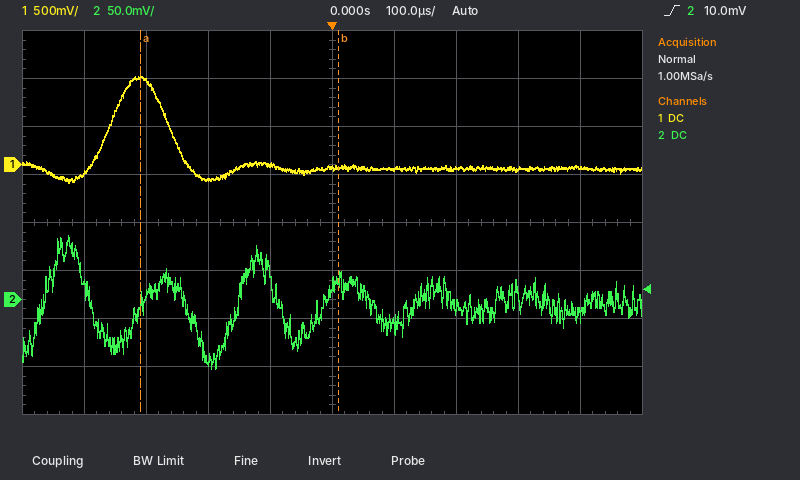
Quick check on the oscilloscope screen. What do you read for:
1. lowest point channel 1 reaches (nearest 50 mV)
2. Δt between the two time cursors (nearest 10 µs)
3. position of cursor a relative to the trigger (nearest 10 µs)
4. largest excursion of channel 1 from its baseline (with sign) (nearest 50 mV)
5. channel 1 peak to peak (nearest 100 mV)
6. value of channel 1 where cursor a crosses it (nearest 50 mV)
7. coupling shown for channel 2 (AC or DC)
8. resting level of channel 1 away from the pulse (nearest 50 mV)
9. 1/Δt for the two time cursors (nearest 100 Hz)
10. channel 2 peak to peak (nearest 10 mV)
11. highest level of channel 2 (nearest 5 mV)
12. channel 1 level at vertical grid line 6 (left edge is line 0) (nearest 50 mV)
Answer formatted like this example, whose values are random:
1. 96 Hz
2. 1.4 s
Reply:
1. -200 mV
2. 320 µs
3. -310 µs
4. +950 mV
5. 1.10 V
6. 900 mV
7. DC
8. -50 mV
9. 3.1 kHz
10. 140 mV
11. 65 mV
12. -50 mV
